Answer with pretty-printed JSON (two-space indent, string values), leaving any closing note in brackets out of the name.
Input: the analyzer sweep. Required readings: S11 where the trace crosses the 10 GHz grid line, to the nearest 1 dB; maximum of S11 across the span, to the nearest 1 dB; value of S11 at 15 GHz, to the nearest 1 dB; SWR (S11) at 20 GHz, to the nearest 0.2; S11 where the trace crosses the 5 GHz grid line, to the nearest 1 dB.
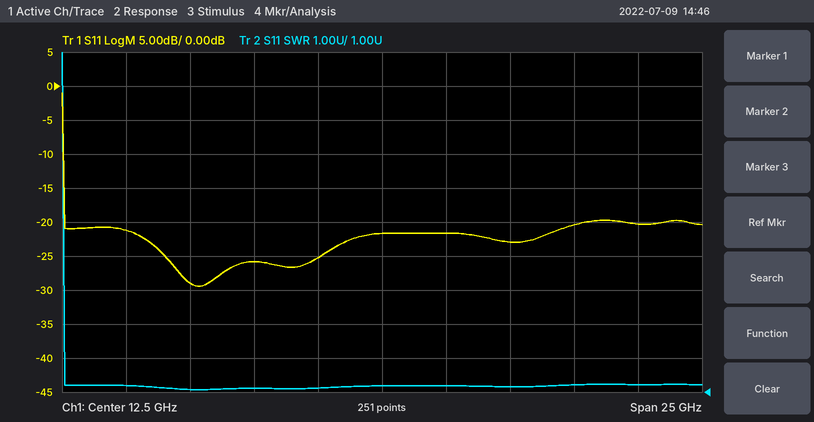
{
  "S11 where the trace crosses the 10 GHz grid line, to the nearest 1 dB": "-25 dB",
  "maximum of S11 across the span, to the nearest 1 dB": "-1 dB",
  "value of S11 at 15 GHz, to the nearest 1 dB": "-22 dB",
  "SWR (S11) at 20 GHz, to the nearest 0.2": "1.2",
  "S11 where the trace crosses the 5 GHz grid line, to the nearest 1 dB": "-29 dB"
}
